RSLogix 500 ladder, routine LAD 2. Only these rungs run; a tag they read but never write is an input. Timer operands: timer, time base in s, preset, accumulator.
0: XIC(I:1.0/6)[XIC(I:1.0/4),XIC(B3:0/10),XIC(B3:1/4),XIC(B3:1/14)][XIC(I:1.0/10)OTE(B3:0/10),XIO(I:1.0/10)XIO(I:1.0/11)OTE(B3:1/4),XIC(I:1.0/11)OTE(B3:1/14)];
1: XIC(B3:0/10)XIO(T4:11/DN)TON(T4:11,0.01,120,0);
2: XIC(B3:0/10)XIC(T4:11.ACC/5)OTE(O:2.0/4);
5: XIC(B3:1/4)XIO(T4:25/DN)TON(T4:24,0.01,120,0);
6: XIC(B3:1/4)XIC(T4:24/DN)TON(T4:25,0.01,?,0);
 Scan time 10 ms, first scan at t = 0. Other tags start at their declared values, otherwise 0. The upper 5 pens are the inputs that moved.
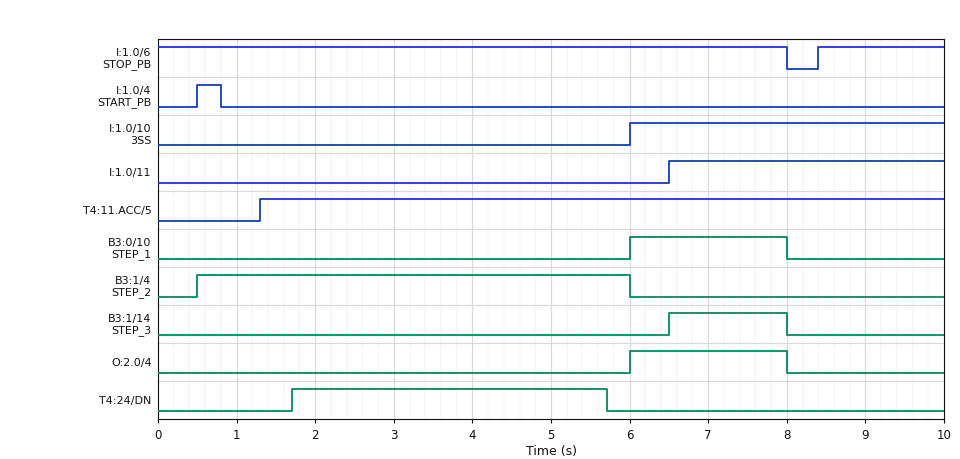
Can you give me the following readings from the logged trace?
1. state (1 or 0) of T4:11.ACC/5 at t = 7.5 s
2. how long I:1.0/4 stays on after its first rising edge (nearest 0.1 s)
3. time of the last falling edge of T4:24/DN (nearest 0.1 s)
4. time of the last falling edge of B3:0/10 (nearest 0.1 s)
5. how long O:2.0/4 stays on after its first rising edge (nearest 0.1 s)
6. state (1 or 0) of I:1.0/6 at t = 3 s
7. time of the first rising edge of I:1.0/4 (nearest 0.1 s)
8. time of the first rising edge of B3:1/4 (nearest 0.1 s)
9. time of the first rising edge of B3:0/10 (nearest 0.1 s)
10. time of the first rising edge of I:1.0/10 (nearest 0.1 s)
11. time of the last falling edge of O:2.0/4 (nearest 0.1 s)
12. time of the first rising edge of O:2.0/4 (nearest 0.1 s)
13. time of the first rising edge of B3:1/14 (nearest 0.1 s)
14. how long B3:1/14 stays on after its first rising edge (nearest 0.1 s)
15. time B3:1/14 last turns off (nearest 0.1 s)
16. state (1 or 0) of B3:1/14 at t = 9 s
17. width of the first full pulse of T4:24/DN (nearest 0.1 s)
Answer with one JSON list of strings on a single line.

["1", "0.3 s", "5.7 s", "8.0 s", "2.0 s", "1", "0.5 s", "0.5 s", "6.0 s", "6.0 s", "8.0 s", "6.0 s", "6.5 s", "1.5 s", "8.0 s", "0", "4.0 s"]
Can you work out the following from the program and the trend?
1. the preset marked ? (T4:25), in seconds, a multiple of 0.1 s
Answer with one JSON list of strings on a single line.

["4.0 s"]
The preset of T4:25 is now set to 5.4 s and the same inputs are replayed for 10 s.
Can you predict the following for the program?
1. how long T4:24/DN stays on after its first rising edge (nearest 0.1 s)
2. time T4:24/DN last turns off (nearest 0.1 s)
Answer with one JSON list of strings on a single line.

["4.3 s", "6.0 s"]
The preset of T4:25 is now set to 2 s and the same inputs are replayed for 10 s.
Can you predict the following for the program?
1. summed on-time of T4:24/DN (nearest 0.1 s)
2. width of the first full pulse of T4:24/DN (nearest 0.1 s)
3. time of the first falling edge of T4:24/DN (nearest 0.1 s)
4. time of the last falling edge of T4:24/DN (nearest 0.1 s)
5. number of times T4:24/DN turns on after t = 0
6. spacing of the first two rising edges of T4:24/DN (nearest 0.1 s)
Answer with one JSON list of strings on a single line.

["3.1 s", "2.0 s", "3.7 s", "6.0 s", "2", "3.2 s"]
